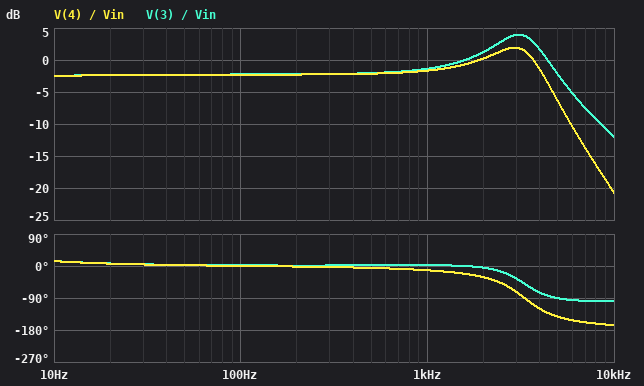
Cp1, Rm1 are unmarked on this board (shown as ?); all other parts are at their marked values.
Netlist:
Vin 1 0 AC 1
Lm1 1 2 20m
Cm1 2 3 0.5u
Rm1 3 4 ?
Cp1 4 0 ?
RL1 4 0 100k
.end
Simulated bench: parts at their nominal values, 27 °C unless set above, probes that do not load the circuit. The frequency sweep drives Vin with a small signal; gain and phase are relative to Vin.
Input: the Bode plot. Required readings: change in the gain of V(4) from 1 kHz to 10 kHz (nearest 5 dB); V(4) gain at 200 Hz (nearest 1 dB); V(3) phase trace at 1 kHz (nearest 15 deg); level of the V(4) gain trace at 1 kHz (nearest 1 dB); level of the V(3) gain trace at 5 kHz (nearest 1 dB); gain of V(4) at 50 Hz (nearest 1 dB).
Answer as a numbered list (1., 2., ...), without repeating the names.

1. -20 dB
2. -2 dB
3. 0 deg
4. -2 dB
5. -2 dB
6. -2 dB
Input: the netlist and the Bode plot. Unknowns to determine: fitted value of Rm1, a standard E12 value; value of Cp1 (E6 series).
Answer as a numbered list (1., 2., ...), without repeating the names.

1. 270 Ω
2. 150 nF
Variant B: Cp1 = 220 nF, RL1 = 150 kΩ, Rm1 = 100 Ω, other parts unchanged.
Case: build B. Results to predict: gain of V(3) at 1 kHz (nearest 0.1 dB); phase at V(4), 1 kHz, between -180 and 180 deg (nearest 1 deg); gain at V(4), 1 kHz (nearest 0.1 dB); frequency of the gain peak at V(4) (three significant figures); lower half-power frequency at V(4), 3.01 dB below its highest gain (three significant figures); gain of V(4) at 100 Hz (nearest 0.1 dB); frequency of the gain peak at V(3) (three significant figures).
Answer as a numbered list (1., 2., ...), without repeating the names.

1. -2.0 dB
2. -6 deg
3. -2.1 dB
4. 2.82 kHz
5. 2.39 kHz
6. -3.2 dB
7. 2.83 kHz
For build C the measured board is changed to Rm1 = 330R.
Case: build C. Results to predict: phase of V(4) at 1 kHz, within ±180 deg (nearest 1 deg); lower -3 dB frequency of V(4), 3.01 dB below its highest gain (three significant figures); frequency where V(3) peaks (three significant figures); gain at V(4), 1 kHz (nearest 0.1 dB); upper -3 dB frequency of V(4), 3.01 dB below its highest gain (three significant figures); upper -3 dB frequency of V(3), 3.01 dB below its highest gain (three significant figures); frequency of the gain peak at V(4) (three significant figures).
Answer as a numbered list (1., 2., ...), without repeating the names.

1. -15 deg
2. 9.75 Hz
3. 3.04 kHz
4. -1.8 dB
5. 3.94 kHz
6. 4.40 kHz
7. 2.74 kHz
